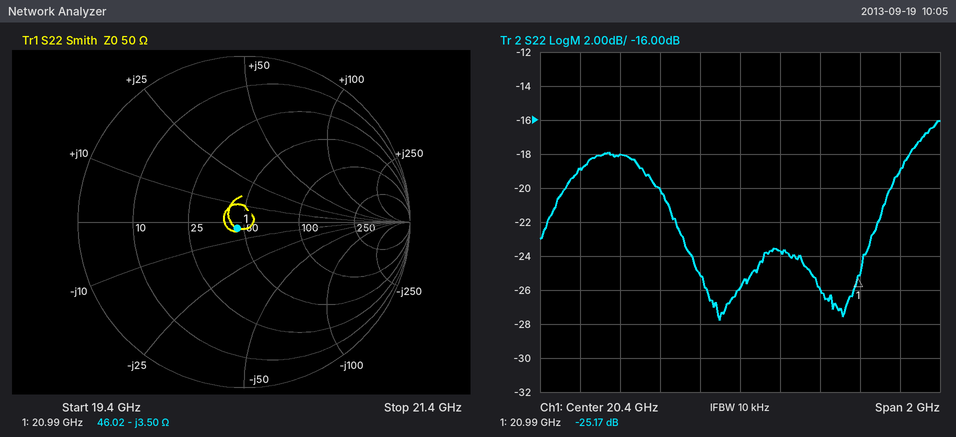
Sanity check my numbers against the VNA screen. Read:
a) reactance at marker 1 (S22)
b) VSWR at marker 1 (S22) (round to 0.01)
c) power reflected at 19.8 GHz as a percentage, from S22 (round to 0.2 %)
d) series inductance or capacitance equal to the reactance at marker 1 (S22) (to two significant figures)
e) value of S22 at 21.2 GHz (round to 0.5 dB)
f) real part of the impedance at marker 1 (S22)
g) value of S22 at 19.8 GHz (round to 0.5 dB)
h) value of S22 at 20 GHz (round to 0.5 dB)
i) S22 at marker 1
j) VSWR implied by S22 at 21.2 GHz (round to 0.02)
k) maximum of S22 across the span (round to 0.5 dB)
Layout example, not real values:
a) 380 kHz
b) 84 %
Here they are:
a) -3.50 Ω
b) 1.12
c) 1.6 %
d) 2.2 pF
e) -19.0 dB
f) 46.02 Ω
g) -18.0 dB
h) -20.0 dB
i) -25.17 dB
j) 1.26
k) -16.0 dB
